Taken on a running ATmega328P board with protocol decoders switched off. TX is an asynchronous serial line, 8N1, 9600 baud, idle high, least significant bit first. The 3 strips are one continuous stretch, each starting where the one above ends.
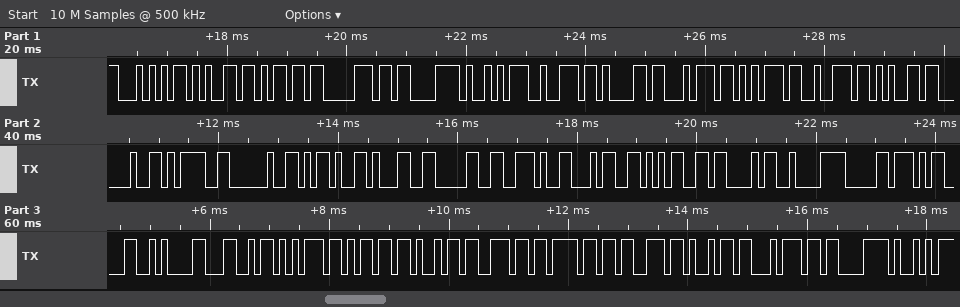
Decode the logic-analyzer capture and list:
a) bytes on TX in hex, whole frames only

0x54 0x65 0x6D 0x70 0xC3 0xA9 0x72 0x61 0x74 0x75 0x72 0x65 0x20 0x3D 0x20 0x2D 0x31 0x30 0x2E 0x34 0x35 0x43 0xC2 0xB0 0x0D 0x0A 0x4C 0x75 0x6D 0x69 0x6E 0x6F 0x73 0x69 0x74 0xC3 0xA9
